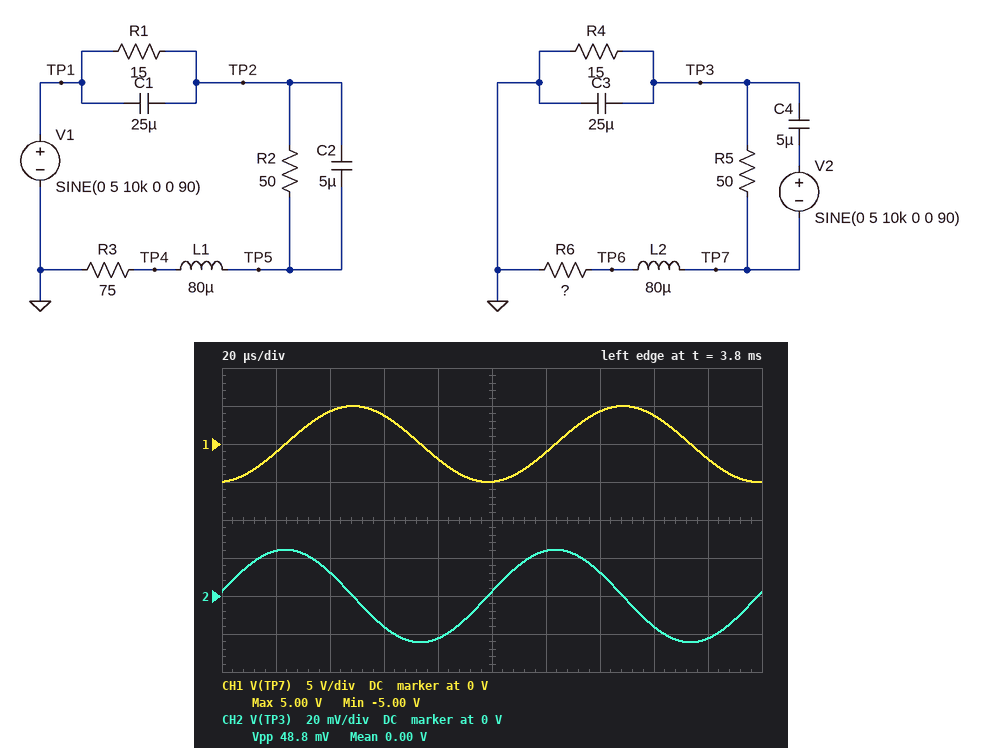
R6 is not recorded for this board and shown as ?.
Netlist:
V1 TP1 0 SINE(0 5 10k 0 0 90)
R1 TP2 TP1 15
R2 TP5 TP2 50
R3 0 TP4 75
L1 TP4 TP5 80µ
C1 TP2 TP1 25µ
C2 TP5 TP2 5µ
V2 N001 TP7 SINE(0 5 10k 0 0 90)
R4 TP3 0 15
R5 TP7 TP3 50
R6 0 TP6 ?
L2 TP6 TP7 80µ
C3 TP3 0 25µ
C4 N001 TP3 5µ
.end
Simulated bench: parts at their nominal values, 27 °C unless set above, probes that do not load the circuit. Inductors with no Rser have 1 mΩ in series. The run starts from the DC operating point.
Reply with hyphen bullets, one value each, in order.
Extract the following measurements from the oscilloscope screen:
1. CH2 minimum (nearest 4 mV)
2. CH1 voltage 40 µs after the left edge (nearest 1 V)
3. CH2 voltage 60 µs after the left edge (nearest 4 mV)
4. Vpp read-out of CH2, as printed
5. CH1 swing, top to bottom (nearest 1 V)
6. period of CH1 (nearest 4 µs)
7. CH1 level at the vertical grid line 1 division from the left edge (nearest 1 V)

- -24 mV
- 4 V
- -16 mV
- 48.8 mV
- 10 V
- 100 µs
- -1 V
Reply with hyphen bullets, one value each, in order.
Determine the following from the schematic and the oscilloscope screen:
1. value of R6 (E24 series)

- 130 Ω
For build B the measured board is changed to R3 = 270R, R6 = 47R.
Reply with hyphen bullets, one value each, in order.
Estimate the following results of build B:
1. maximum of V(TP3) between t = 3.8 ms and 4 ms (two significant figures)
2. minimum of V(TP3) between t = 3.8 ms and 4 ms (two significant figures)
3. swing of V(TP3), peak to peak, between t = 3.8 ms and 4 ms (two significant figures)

- 67 mV
- -67 mV
- 130 mV
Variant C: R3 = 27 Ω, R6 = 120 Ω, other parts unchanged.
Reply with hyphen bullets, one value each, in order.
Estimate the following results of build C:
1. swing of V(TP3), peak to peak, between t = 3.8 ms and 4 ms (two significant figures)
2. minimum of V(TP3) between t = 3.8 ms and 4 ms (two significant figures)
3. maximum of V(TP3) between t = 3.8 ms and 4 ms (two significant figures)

- 53 mV
- -26 mV
- 26 mV
